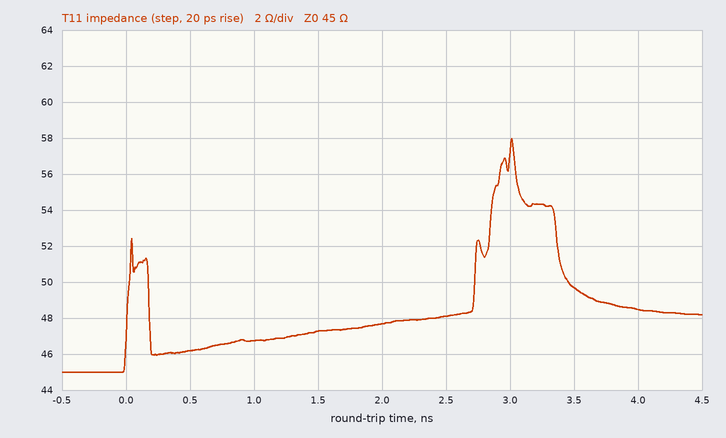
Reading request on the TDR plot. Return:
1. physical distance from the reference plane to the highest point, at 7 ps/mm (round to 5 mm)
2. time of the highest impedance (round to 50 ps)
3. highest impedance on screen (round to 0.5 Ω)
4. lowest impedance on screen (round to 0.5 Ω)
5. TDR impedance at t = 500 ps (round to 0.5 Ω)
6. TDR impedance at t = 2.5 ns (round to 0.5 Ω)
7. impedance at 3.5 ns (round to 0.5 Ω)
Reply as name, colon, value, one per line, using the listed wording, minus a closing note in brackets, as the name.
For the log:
physical distance from the reference plane to the highest point, at 7 ps/mm: 215 mm
time of the highest impedance: 3.00 ns
highest impedance on screen: 58.0 Ω
lowest impedance on screen: 45.0 Ω
TDR impedance at t = 500 ps: 46.0 Ω
TDR impedance at t = 2.5 ns: 48.0 Ω
impedance at 3.5 ns: 49.5 Ω
